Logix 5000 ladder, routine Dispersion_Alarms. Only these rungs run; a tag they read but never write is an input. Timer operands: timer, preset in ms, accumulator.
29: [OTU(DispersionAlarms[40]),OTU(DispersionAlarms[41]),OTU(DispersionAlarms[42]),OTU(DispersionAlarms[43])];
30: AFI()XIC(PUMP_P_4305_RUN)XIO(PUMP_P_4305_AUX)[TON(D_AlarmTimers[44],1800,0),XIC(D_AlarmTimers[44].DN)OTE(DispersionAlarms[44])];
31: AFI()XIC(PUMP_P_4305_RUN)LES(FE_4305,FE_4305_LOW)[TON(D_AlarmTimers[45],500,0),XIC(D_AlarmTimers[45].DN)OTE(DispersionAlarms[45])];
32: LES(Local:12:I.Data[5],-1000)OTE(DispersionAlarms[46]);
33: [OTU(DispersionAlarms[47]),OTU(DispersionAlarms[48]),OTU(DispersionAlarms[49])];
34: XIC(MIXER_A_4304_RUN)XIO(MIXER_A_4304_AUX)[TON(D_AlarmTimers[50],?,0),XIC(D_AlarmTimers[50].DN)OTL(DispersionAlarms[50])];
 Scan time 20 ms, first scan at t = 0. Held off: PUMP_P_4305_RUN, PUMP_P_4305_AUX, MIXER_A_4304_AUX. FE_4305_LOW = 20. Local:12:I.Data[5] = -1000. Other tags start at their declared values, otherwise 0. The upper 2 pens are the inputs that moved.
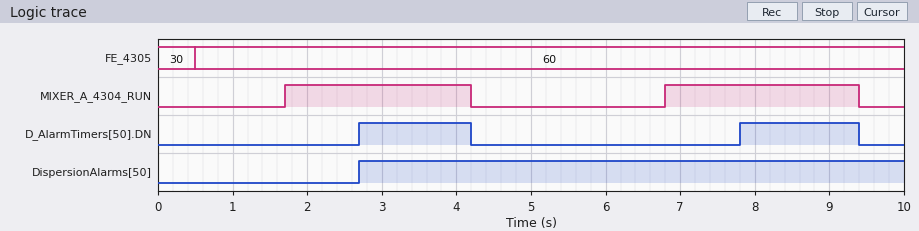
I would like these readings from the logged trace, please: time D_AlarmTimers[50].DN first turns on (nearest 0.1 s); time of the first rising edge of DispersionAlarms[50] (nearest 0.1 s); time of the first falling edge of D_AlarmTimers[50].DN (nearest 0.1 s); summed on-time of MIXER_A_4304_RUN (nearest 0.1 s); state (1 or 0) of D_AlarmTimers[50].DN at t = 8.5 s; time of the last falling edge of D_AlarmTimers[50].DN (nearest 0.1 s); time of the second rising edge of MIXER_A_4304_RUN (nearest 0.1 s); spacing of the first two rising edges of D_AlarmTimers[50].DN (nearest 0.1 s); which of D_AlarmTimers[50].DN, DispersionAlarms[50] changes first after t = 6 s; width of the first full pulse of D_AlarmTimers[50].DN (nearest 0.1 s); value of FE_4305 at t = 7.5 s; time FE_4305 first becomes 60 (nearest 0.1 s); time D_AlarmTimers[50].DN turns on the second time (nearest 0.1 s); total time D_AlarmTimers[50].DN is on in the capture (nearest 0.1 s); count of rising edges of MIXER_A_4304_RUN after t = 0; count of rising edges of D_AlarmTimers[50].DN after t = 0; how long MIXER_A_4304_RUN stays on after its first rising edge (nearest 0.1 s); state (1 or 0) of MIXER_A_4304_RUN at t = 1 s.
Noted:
2.7 s
2.7 s
4.2 s
5.1 s
1
9.4 s
6.8 s
5.1 s
D_AlarmTimers[50].DN
1.5 s
60
0.5 s
7.8 s
3.1 s
2
2
2.5 s
0
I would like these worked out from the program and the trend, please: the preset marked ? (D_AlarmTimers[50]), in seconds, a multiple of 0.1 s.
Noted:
1.0 s
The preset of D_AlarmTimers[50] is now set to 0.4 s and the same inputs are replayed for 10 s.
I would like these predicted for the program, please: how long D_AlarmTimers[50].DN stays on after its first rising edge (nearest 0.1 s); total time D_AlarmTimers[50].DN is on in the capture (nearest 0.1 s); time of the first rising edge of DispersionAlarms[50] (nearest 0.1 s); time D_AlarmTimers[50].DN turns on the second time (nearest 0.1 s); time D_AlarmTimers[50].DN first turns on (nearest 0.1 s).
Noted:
2.1 s
4.3 s
2.1 s
7.2 s
2.1 s
